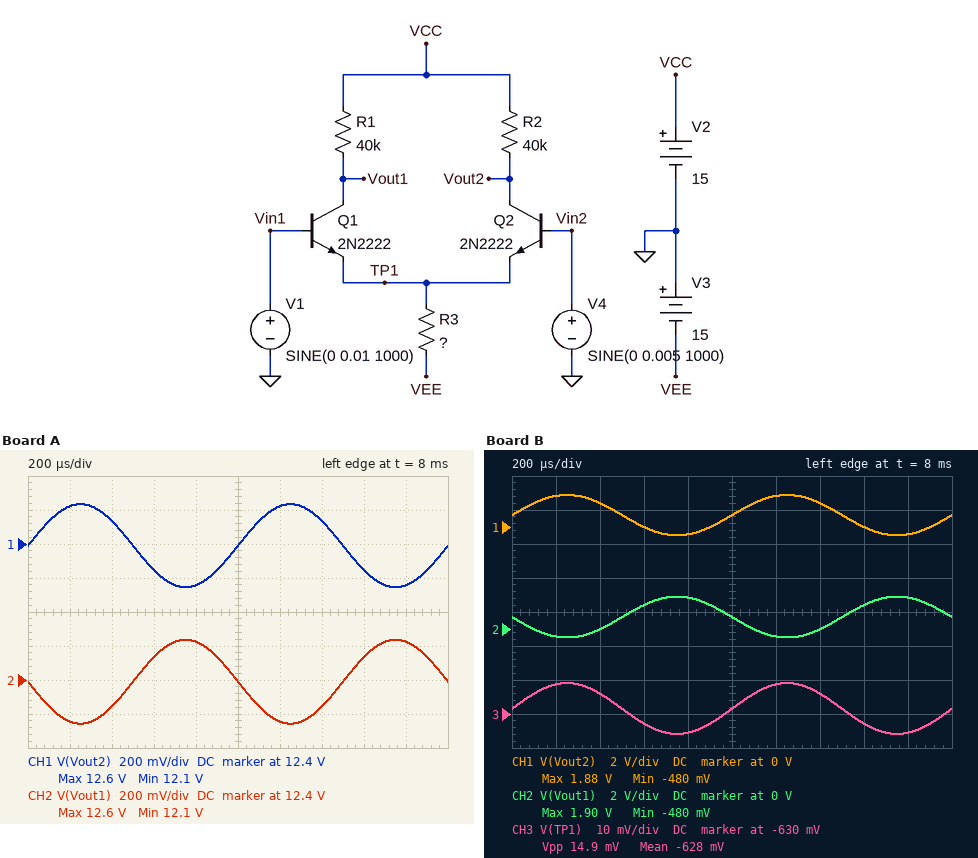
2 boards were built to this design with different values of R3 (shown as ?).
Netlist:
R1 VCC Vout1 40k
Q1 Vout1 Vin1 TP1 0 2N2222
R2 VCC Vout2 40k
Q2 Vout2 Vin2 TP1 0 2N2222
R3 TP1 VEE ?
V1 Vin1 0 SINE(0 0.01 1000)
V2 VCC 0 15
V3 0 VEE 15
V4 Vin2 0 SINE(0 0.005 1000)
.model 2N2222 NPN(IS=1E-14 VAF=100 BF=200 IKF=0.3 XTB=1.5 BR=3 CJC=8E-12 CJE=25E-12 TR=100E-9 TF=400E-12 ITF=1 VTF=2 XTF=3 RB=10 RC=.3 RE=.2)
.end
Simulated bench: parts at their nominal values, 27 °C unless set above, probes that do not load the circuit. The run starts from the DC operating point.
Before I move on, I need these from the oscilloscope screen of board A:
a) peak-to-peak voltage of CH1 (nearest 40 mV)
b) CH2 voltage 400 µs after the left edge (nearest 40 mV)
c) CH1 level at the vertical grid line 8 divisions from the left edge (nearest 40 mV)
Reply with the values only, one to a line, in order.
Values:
480 mV
12.24 V
12.24 V
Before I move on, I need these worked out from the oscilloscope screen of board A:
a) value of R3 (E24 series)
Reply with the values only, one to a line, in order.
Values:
110 kΩ
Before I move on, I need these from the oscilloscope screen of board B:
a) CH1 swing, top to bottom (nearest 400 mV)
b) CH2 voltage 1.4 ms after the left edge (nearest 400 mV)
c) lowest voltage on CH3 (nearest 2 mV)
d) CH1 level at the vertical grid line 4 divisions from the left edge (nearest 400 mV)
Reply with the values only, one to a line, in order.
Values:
2.4 V
0 V
-636 mV
-400 mV
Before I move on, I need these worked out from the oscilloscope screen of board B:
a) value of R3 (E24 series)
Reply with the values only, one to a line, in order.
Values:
20 kΩ
